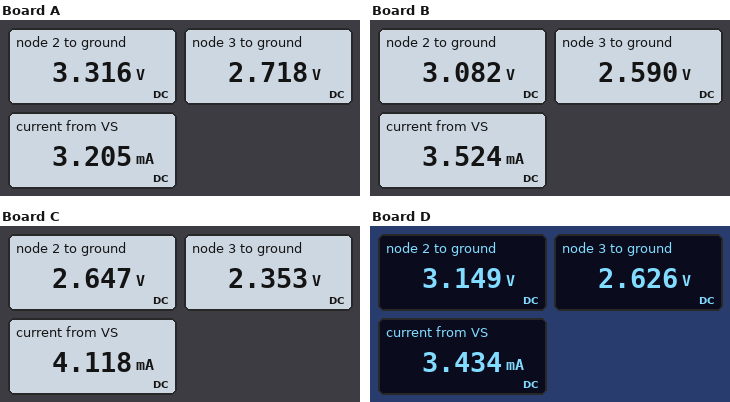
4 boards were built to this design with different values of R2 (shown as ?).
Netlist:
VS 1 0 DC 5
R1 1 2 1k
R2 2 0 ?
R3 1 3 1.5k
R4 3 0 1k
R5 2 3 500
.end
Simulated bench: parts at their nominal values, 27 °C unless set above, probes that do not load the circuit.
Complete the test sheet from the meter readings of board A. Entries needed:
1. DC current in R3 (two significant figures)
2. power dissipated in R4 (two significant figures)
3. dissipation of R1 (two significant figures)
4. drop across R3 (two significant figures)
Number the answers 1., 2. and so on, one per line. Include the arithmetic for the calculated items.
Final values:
1. (5 V - 2.718 V) / 1.5 kΩ = 1.5 mA
2. (2.718 V)^2 / 1 kΩ = 7.4 mW
3. (5 V - 3.316 V)^2 / 1 kΩ = 2.8 mW
4. 5 V - 2.718 V = 2.3 V
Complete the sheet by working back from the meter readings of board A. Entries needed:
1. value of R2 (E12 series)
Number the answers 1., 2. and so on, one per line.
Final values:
1. 6.8 kΩ
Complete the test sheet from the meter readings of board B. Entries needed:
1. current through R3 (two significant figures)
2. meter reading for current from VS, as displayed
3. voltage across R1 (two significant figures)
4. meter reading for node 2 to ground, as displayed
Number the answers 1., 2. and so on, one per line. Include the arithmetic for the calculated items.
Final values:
1. (5 V - 2.59 V) / 1.5 kΩ = 1.6 mA
2. 3.524 mA
3. 5 V - 3.082 V = 1.9 V
4. 3.082 V
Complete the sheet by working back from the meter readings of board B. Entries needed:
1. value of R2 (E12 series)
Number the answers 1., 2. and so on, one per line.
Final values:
1. 3.3 kΩ
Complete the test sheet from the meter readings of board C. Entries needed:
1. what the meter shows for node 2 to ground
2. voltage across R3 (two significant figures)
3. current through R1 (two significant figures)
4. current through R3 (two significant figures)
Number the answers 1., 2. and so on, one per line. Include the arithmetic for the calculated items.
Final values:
1. 2.647 V
2. 5 V - 2.353 V = 2.6 V
3. (5 V - 2.647 V) / 1 kΩ = 2.4 mA
4. (5 V - 2.353 V) / 1.5 kΩ = 1.8 mA
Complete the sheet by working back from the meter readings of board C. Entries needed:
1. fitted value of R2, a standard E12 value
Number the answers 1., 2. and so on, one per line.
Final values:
1. 1.5 kΩ
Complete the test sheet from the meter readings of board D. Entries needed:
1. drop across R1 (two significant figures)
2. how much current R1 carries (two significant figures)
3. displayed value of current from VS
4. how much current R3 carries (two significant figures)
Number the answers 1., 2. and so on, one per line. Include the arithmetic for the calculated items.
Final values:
1. 5 V - 3.149 V = 1.9 V
2. (5 V - 3.149 V) / 1 kΩ = 1.9 mA
3. 3.434 mA
4. (5 V - 2.626 V) / 1.5 kΩ = 1.6 mA
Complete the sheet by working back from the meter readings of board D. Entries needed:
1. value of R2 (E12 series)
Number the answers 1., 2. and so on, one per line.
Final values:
1. 3.9 kΩ
